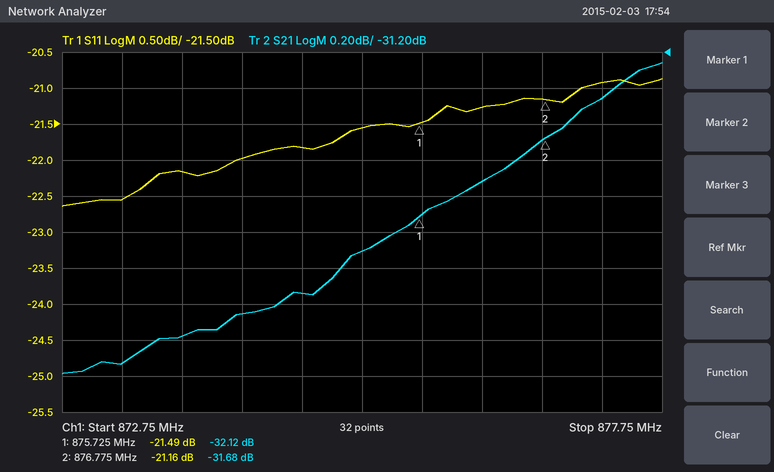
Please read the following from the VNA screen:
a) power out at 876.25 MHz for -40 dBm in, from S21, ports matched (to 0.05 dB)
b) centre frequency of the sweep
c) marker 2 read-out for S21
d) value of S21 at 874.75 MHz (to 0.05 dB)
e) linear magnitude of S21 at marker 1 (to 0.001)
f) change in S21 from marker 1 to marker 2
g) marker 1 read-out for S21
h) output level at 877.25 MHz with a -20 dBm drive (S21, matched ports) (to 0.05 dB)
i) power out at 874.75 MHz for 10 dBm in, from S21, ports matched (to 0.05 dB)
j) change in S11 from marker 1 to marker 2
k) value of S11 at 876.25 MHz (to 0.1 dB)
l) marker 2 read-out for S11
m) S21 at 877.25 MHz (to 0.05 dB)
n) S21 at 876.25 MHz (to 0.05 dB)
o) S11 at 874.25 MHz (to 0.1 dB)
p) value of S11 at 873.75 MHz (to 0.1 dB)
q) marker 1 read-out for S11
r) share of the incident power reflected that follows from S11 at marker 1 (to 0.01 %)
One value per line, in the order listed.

-71.90 dBm
875.25 MHz
-31.68 dB
-32.55 dB
0.025
0.44 dB
-32.12 dB
-51.45 dBm
-22.55 dBm
0.33 dB
-21.3 dB
-21.16 dB
-31.45 dB
-31.90 dB
-22.0 dB
-22.2 dB
-21.49 dB
0.71 %
